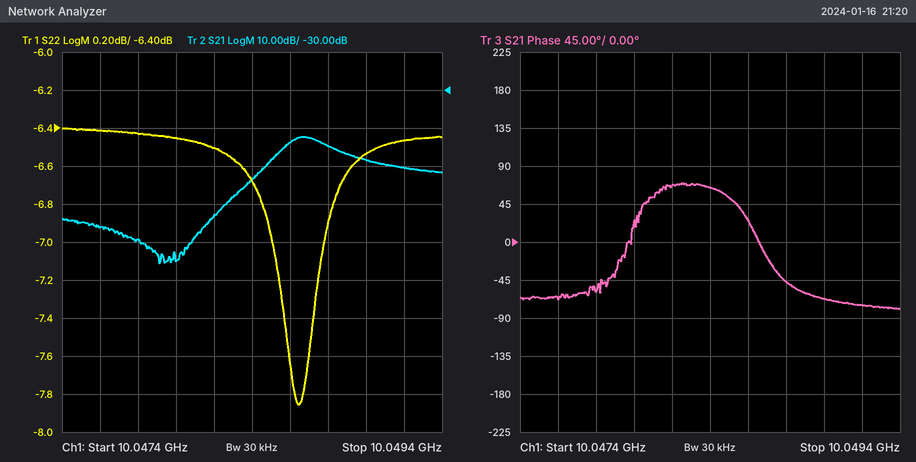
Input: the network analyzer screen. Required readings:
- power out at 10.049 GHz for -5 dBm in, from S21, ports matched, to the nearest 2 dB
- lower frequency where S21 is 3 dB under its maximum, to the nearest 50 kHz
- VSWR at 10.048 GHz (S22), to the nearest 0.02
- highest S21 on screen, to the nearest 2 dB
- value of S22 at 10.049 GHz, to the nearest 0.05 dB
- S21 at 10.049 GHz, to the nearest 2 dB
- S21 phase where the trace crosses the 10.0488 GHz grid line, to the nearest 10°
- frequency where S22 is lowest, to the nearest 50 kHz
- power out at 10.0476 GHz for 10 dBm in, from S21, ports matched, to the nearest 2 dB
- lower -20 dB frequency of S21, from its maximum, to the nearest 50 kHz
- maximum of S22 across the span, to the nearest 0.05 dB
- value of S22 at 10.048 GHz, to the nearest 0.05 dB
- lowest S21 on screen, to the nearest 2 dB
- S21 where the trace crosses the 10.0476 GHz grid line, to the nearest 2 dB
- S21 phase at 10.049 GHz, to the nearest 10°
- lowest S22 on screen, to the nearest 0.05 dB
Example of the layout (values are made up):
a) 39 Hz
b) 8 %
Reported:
a) -54 dBm
b) 10.04855 GHz
c) 2.82
d) -42 dB
e) -6.55 dB
f) -48 dB
g) -50°
h) 10.04865 GHz
i) -56 dBm
j) 10.04820 GHz
k) -6.40 dB
l) -6.45 dB
m) -76 dB
n) -66 dB
o) -70°
p) -7.85 dB
